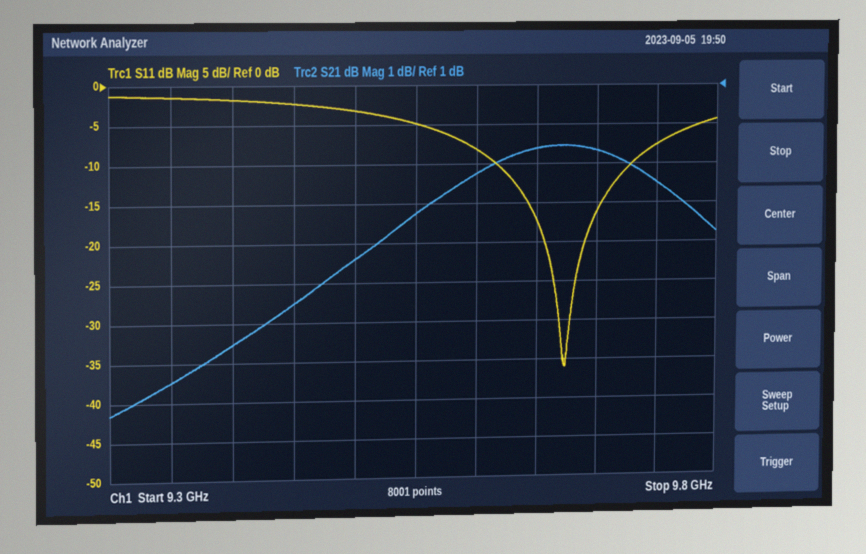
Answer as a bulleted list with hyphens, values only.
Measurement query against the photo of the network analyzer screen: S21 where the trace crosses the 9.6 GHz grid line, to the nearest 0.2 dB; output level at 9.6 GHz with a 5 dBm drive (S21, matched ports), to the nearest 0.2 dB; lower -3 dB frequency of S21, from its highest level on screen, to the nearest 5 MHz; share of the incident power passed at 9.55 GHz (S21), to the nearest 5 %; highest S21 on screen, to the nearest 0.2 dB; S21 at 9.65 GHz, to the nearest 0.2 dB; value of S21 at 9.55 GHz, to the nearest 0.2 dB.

- -1.2 dB
- 3.8 dBm
- 9.495 GHz
- 60 %
- -0.6 dB
- -0.6 dB
- -2.2 dB
